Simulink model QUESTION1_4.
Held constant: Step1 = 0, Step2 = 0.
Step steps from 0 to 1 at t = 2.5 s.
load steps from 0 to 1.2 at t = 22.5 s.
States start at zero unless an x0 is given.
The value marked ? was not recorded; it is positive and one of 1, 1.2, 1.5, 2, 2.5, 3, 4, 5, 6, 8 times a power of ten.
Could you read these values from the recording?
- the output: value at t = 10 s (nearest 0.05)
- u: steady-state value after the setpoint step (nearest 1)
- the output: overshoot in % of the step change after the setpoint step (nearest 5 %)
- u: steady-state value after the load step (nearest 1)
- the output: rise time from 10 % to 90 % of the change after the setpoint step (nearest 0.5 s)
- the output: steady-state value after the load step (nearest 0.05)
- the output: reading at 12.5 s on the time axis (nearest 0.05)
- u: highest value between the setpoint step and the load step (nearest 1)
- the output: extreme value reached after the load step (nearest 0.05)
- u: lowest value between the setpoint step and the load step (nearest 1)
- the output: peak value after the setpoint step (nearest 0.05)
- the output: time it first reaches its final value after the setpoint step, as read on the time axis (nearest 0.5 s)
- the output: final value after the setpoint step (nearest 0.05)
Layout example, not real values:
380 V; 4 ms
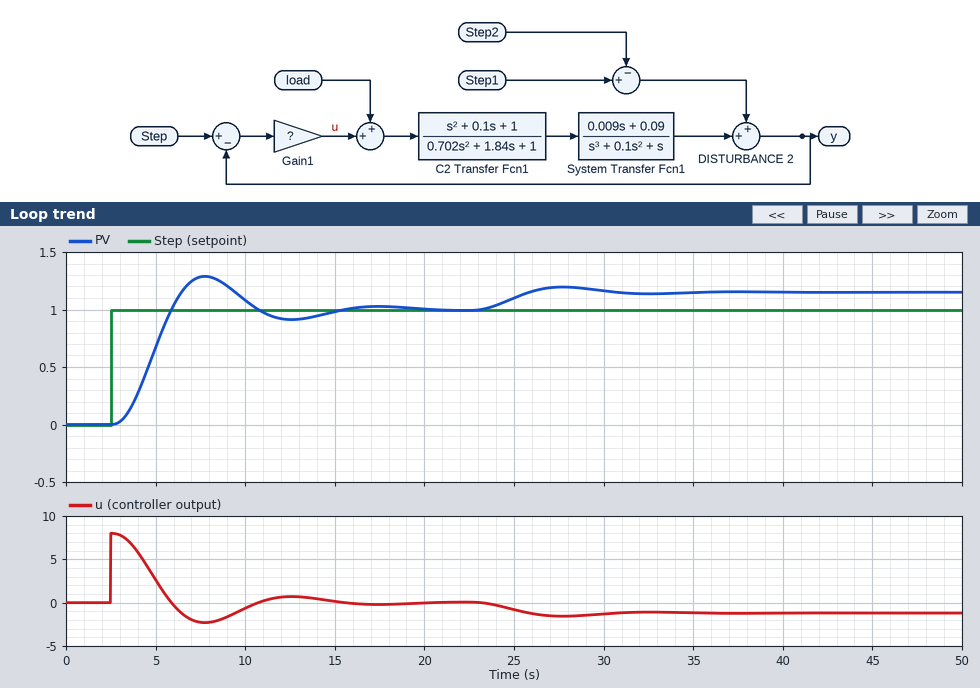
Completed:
1.10; 0; 30 %; -1; 2.0 s; 1.15; 0.90; 8; 1.20; -2; 1.30; 6.0 s; 1.00
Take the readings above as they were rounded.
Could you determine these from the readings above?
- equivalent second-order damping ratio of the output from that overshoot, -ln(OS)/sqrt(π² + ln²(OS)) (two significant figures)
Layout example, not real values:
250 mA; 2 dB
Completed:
0.36
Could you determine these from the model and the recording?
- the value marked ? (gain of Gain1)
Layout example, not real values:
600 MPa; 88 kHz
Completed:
8
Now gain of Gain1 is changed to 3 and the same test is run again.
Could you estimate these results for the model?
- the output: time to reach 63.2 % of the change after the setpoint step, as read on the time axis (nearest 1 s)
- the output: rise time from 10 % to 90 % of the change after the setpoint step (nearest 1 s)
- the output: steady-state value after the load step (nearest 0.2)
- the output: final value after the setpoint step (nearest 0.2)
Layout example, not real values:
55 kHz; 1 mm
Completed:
7 s; 5 s; 1.4; 1.0
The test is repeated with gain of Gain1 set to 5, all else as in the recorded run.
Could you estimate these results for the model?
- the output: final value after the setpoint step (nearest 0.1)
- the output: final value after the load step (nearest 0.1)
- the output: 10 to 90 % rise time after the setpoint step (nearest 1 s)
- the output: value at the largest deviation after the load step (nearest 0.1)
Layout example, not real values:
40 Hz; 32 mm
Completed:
1.0; 1.2; 3 s; 1.3
